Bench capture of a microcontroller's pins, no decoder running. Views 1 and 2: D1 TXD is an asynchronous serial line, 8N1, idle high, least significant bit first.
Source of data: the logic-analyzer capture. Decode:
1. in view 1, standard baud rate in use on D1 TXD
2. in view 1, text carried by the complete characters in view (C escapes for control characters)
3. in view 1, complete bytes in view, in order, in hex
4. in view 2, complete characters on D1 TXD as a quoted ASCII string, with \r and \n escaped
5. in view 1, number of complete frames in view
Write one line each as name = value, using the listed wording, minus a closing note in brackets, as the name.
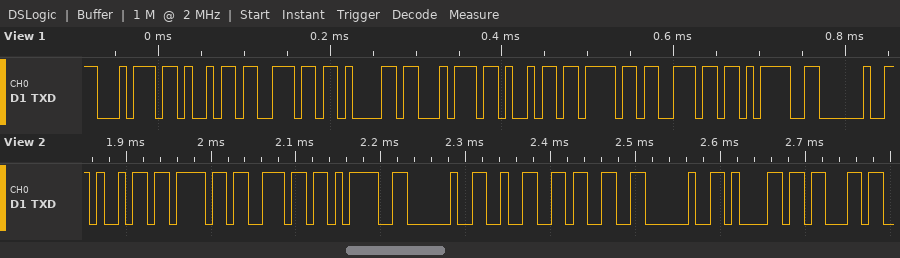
in view 1, standard baud rate in use on D1 TXD = 115200 baud
in view 1, text carried by the complete characters in view = "tination= "
in view 1, complete bytes in view, in order, in hex = 74 69 6E 61 74 69 6F 6E 3D 20
in view 2, complete characters on D1 TXD as a quoted ASCII string, with \r and \n escaped = "ion= 23 ac"
in view 1, number of complete frames in view = 10
